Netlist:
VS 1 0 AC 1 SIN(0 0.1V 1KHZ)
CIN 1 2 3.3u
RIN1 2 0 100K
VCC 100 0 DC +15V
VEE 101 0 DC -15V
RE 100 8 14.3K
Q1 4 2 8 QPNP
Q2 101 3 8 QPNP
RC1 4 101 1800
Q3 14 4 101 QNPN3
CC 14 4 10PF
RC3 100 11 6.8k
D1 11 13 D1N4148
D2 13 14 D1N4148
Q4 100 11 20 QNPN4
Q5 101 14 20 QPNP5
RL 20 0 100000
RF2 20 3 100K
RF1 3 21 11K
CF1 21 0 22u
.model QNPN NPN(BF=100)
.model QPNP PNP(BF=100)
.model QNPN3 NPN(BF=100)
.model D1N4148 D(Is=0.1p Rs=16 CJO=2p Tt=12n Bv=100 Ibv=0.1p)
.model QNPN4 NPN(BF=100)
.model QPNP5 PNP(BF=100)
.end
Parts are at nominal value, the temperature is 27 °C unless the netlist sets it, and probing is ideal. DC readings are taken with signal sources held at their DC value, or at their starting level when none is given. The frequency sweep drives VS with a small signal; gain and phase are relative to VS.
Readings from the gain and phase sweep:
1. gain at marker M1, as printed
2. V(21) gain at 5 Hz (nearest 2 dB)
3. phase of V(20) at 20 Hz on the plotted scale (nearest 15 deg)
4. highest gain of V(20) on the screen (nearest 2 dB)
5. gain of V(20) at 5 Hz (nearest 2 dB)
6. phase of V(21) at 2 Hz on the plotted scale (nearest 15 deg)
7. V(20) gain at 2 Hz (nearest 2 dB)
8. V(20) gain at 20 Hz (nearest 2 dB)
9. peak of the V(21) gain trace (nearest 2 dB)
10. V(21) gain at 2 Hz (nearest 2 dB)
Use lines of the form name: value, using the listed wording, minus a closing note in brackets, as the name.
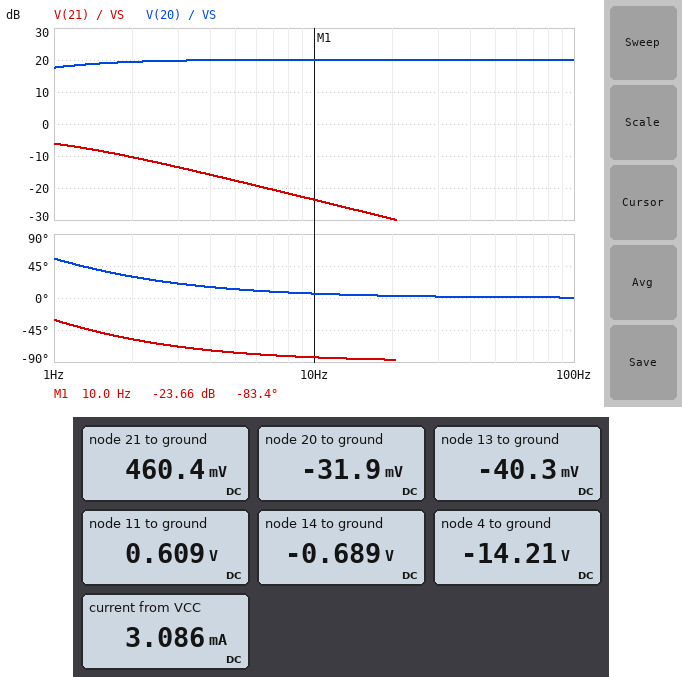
gain at marker M1, as printed: -23.66 dB
V(21) gain at 5 Hz: -18 dB
phase of V(20) at 20 Hz on the plotted scale: 0 deg
highest gain of V(20) on the screen: 20 dB
gain of V(20) at 5 Hz: 20 dB
phase of V(21) at 2 Hz on the plotted scale: -60 deg
V(20) gain at 2 Hz: 20 dB
V(20) gain at 20 Hz: 20 dB
peak of the V(21) gain trace: -6 dB
V(21) gain at 2 Hz: -10 dB
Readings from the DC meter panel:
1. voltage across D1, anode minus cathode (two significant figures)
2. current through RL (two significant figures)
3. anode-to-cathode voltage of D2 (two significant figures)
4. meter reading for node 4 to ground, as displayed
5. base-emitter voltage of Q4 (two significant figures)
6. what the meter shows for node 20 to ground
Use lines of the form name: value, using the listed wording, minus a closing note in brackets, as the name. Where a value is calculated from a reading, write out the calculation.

voltage across D1, anode minus cathode: 609 mV - (-40.3 mV) = 650 mV
current through RL: (0 V - (-31.9 mV)) / 100 kΩ = 320 nA
anode-to-cathode voltage of D2: -40.3 mV - (-689 mV) = 650 mV
meter reading for node 4 to ground, as displayed: -14.21 V
base-emitter voltage of Q4: 609 mV - (-31.9 mV) = 640 mV
what the meter shows for node 20 to ground: -31.9 mV
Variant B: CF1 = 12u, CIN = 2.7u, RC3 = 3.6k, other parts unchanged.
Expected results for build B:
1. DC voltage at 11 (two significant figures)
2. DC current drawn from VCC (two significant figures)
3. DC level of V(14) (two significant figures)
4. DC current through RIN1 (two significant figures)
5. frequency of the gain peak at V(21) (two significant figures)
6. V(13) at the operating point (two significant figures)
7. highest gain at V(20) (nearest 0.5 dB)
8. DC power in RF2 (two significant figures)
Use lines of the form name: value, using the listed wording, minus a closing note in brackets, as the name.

DC voltage at 11: 720 mV
DC current drawn from VCC: 5.0 mA
DC level of V(14): -670 mV
DC current through RIN1: 4.9 µA
frequency of the gain peak at V(21): 840 mHz
V(13) at the operating point: 27 mV
highest gain at V(20): 20.0 dB
DC power in RF2: 2.1 µW
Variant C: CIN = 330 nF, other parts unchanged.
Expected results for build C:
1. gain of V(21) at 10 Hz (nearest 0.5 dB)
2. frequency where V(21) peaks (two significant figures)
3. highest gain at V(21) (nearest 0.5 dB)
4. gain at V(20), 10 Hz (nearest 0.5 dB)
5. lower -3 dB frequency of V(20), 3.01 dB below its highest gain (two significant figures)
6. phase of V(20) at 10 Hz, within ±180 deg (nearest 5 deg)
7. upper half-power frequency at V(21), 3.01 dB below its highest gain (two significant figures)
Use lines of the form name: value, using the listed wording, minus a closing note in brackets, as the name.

gain of V(21) at 10 Hz: -24.5 dB
frequency where V(21) peaks: 1.8 Hz
highest gain at V(21): -18.5 dB
gain at V(20), 10 Hz: 19.0 dB
lower -3 dB frequency of V(20), 3.01 dB below its highest gain: 5.0 Hz
phase of V(20) at 10 Hz, within ±180 deg: 30 deg
upper half-power frequency at V(21), 3.01 dB below its highest gain: 6.1 Hz
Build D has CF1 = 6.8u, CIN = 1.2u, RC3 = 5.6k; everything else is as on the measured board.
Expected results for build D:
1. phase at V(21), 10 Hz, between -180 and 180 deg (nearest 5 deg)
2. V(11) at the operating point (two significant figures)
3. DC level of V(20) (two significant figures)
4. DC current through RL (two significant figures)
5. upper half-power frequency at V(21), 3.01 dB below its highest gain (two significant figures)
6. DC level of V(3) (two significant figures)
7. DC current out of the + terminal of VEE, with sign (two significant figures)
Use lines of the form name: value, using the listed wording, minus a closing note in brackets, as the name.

phase at V(21), 10 Hz, between -180 and 180 deg: -70 deg
V(11) at the operating point: 640 mV
DC level of V(20): -16 mV
DC current through RL: 160 nA
upper half-power frequency at V(21), 3.01 dB below its highest gain: 4.2 Hz
DC level of V(3): 470 mV
DC current out of the + terminal of VEE, with sign: -3.5 mA
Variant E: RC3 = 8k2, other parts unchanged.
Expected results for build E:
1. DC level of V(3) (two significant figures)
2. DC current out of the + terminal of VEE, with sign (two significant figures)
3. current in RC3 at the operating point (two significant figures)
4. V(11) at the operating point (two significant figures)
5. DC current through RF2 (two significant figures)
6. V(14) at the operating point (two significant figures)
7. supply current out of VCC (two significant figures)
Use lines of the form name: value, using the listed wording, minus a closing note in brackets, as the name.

DC level of V(3): 450 mV
DC current out of the + terminal of VEE, with sign: -2.7 mA
current in RC3 at the operating point: 1.8 mA
V(11) at the operating point: 580 mV
DC current through RF2: 5.0 µA
V(14) at the operating point: -700 mV
supply current out of VCC: 2.7 mA
